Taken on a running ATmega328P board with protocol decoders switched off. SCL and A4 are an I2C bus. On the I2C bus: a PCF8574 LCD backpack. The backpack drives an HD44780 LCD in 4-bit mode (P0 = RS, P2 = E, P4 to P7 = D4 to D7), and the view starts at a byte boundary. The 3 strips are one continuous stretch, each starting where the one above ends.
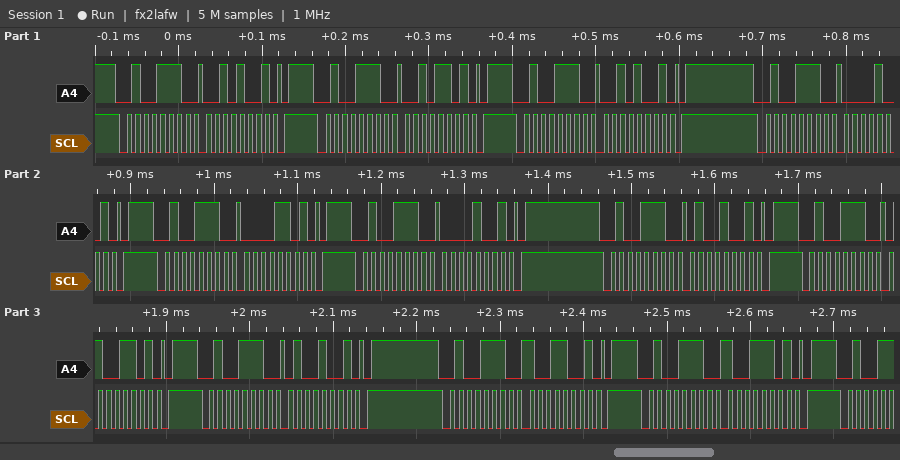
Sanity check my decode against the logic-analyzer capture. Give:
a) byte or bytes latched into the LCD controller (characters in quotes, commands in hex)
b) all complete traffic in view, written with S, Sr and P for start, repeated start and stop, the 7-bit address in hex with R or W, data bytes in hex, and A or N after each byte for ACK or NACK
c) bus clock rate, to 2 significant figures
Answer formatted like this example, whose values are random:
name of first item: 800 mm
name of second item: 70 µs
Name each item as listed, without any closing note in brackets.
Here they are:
byte or bytes latched into the LCD controller: ' '
all complete traffic in view, written with S, Sr and P for start, repeated start and stop, the 7-bit address in hex with R or W, data bytes in hex, and A or N after each byte for ACK or NACK: S 27W A 29 A P S 27W A 2D A P S 27W A 29 A P S 27W A 09 A P S 27W A 0D A P S 27W A 09 A P S 27W A 49 A P S 27W A 4D A P S 27W A 49 A P S 27W A 99 A P S 27W A 9D A P
bus clock rate, to 2 significant figures: 100 kHz
